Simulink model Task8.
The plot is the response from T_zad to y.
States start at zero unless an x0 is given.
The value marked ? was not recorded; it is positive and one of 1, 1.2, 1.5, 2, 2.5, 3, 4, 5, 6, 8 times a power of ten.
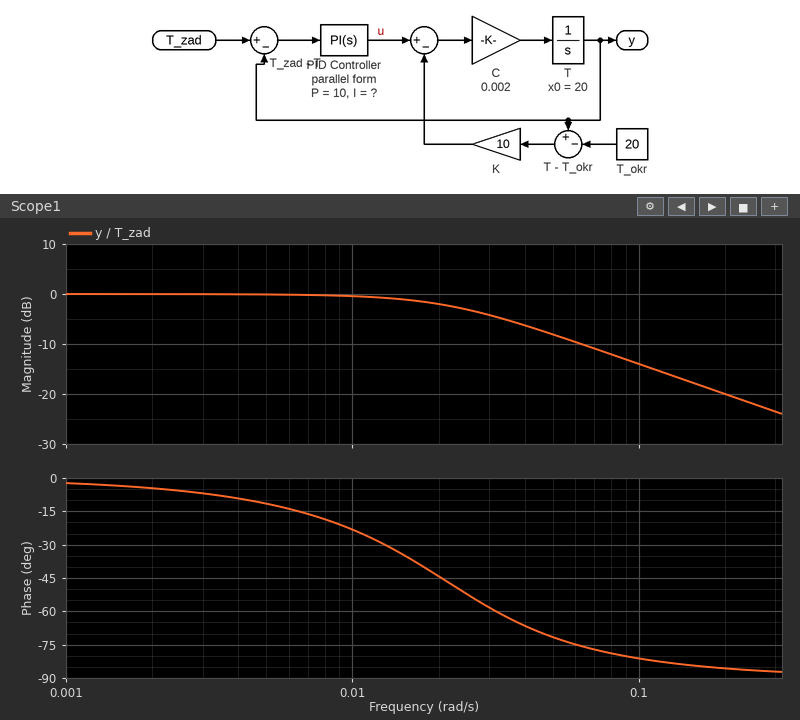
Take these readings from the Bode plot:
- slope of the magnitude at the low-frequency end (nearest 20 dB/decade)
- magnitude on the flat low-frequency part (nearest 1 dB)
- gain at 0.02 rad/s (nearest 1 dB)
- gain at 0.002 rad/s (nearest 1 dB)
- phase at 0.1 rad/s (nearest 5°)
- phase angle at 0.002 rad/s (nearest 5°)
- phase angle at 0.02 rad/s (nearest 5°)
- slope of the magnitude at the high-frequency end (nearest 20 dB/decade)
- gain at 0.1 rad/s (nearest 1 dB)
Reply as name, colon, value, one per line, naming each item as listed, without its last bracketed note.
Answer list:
slope of the magnitude at the low-frequency end: 0 dB/decade
magnitude on the flat low-frequency part: 0 dB
gain at 0.02 rad/s: -2 dB
gain at 0.002 rad/s: 0 dB
phase at 0.1 rad/s: -80°
phase angle at 0.002 rad/s: -5°
phase angle at 0.02 rad/s: -45°
slope of the magnitude at the high-frequency end: -20 dB/decade
gain at 0.1 rad/s: -14 dB
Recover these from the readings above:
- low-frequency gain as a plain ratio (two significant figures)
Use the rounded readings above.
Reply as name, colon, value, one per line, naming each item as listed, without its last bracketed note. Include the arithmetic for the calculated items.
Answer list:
low-frequency gain as a plain ratio: 10^(0 / 20) = 1.0
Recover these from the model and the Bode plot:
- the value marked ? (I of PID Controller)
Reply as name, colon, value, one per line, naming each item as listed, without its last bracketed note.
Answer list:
the value marked ?: 0.25
